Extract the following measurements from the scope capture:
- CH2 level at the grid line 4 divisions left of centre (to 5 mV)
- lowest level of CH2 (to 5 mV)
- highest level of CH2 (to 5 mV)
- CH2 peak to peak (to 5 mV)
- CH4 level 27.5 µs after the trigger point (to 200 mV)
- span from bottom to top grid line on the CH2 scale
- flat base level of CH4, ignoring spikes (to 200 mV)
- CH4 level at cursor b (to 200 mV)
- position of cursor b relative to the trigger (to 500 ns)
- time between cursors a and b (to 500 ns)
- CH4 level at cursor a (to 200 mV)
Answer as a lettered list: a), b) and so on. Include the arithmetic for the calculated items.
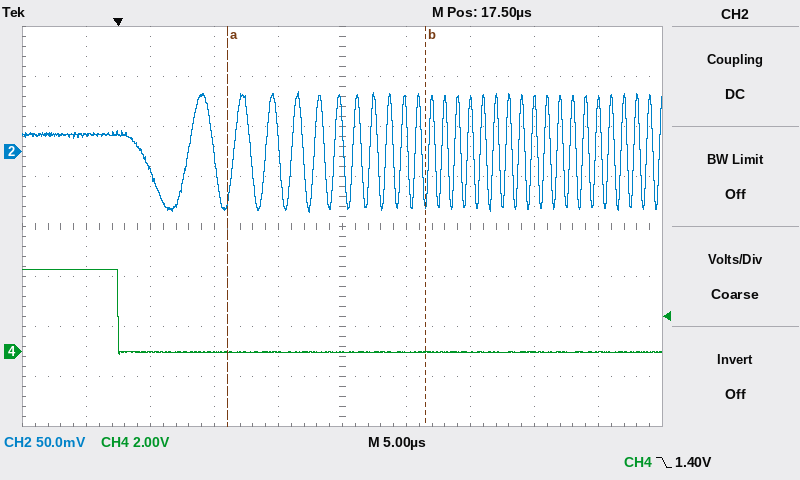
a) 15 mV
b) -60 mV
c) 60 mV
d) 60 mV − (-60 mV) = 120 mV
e) 0.0 V
f) 400 mV
g) 0.0 V
h) 0.0 V
i) +24.0 µs
j) 15.5 µs
k) 0.0 V
